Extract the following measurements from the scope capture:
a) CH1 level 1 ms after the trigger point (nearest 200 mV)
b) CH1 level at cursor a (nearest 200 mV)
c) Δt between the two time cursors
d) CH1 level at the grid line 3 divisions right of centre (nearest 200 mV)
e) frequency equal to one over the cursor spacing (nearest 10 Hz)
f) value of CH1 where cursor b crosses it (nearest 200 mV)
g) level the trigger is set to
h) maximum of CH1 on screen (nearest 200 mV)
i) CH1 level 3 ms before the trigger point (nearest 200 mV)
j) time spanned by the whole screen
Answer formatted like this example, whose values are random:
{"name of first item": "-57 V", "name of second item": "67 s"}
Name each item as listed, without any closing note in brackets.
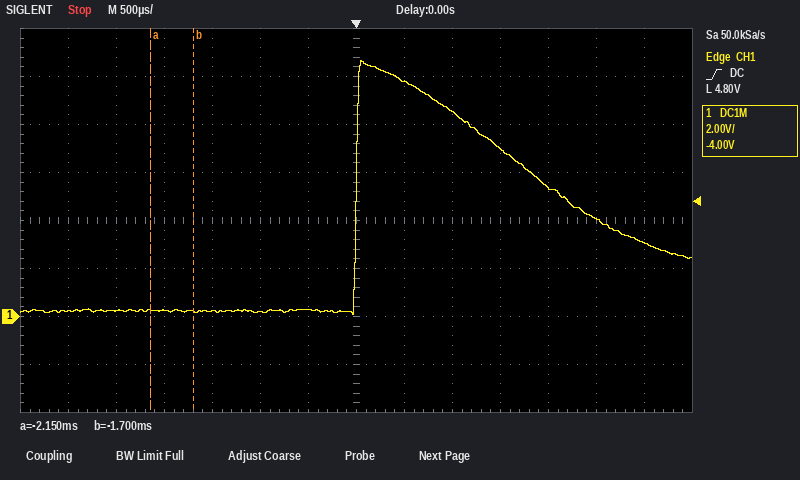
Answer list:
{"CH1 level 1 ms after the trigger point": "8.6 V", "CH1 level at cursor a": "200 mV", "Δt between the two time cursors": "450 µs", "CH1 level at the grid line 3 divisions right of centre": "7.0 V", "frequency equal to one over the cursor spacing": "2.22 kHz", "value of CH1 where cursor b crosses it": "200 mV", "level the trigger is set to": "4.80 V", "maximum of CH1 on screen": "10.6 V", "CH1 level 3 ms before the trigger point": "200 mV", "time spanned by the whole screen": "7 ms"}
